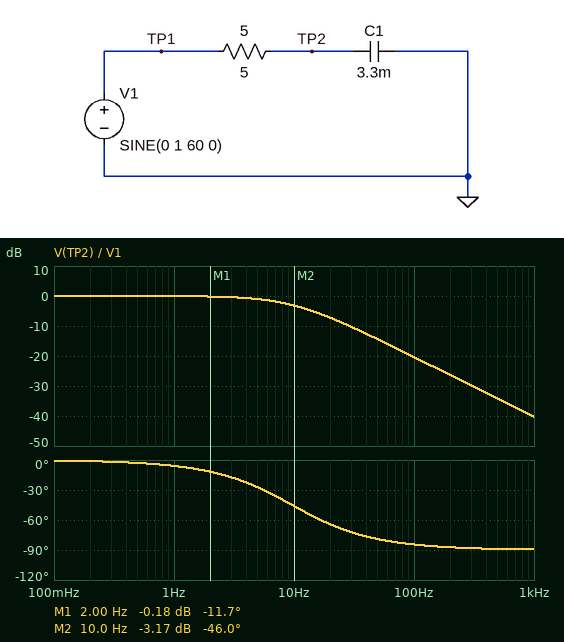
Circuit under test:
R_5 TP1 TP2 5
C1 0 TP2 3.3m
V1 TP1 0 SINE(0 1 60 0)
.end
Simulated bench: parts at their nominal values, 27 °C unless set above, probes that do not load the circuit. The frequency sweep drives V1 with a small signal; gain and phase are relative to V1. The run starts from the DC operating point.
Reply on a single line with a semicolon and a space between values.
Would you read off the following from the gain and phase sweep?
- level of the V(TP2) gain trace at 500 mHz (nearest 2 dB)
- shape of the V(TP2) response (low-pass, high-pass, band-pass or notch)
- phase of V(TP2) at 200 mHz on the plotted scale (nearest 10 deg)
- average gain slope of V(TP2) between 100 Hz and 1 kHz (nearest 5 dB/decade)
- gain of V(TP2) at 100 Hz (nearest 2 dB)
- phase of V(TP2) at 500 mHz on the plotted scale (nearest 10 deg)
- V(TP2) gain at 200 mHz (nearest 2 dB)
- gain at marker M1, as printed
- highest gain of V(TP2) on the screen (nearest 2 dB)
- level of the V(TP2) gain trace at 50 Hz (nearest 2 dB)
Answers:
0 dB; low-pass; 0 deg; -20 dB/decade; -20 dB; 0 deg; 0 dB; -0.18 dB; 0 dB; -14 dB
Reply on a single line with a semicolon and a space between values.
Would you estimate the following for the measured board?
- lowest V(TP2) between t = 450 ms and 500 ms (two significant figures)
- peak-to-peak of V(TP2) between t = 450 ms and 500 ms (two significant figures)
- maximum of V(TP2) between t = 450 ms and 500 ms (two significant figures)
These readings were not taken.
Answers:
-160 mV; 320 mV; 160 mV
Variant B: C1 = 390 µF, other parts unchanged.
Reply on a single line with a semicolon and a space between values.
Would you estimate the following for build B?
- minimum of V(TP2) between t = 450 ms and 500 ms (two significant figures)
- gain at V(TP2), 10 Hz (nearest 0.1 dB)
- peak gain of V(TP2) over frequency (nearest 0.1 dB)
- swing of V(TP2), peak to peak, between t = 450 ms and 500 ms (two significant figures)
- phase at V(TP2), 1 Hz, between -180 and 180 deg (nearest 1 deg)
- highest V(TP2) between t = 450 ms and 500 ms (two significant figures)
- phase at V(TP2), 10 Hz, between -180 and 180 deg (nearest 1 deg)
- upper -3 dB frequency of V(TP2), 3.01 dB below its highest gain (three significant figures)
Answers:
-810 mV; -0.1 dB; 0 dB; 1.6 V; -1 deg; 810 mV; -7 deg; 81.6 Hz
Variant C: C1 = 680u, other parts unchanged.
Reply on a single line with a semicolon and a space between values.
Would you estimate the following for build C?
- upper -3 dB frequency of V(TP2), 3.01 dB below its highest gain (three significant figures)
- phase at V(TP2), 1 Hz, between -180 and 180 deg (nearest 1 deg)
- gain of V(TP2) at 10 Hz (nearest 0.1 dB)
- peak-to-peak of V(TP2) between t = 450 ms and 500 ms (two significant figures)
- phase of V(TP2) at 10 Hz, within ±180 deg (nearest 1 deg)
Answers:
46.8 Hz; -1 deg; -0.2 dB; 1.2 V; -12 deg
